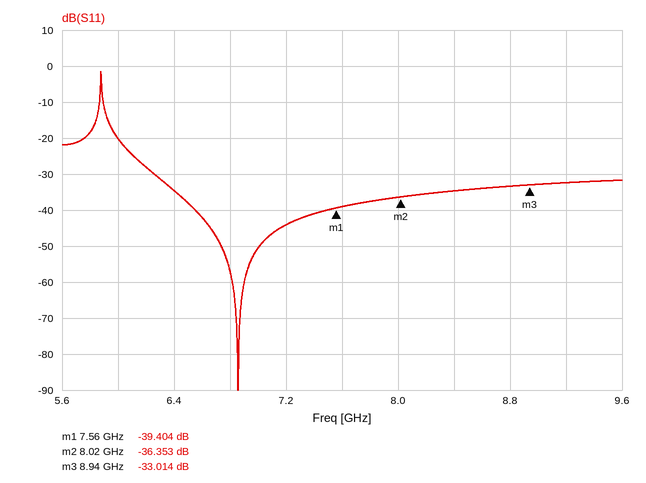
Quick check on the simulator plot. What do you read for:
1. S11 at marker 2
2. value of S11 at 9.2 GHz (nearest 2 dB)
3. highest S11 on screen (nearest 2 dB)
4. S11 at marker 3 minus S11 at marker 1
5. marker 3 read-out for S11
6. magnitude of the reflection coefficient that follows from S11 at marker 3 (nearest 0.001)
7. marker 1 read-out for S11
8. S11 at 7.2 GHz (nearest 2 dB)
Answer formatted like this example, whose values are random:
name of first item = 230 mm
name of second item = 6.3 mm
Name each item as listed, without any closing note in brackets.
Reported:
S11 at marker 2 = -36.353 dB
value of S11 at 9.2 GHz = -32 dB
highest S11 on screen = -2 dB
S11 at marker 3 minus S11 at marker 1 = 6.390 dB
marker 3 read-out for S11 = -33.014 dB
magnitude of the reflection coefficient that follows from S11 at marker 3 = 0.022
marker 1 read-out for S11 = -39.404 dB
S11 at 7.2 GHz = -44 dB
